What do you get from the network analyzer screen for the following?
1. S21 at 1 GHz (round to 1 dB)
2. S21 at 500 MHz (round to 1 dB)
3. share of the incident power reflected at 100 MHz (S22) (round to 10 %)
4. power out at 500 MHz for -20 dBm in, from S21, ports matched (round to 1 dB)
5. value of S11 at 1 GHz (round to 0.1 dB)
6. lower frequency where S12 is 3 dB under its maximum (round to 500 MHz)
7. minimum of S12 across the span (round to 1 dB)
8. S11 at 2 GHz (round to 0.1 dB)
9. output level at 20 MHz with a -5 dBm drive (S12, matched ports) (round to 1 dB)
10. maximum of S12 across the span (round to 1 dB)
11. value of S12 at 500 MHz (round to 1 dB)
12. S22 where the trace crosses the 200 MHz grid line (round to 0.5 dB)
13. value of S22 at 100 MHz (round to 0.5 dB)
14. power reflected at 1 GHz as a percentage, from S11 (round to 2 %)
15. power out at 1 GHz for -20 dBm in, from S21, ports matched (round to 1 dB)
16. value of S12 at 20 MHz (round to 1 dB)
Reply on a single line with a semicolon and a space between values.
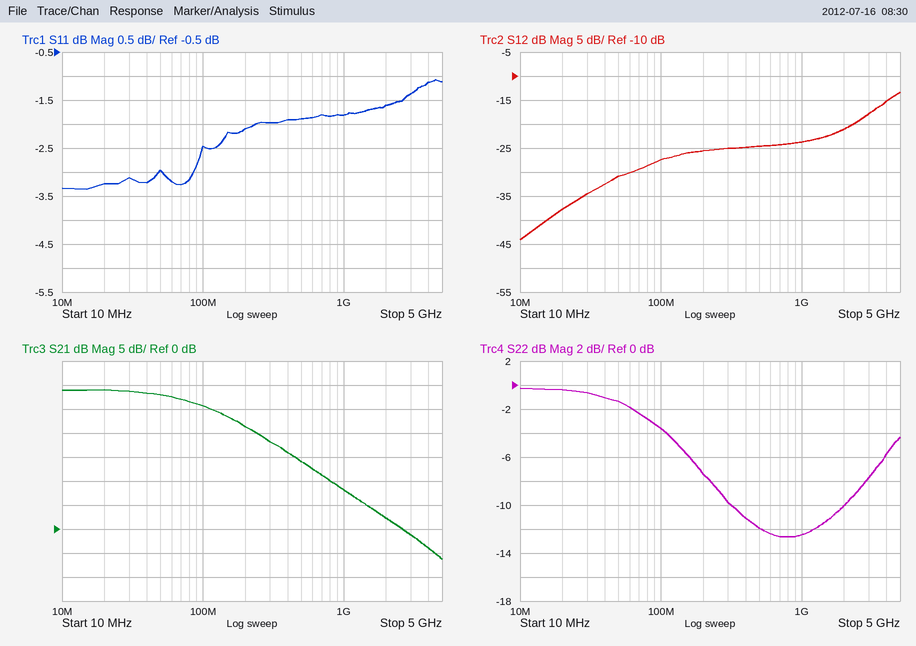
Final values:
8 dB; 14 dB; 40 %; -6 dBm; -1.8 dB; 3.5 GHz; -44 dB; -1.6 dB; -43 dBm; -13 dB; -25 dB; -7.5 dB; -3.5 dB; 66 %; -12 dBm; -38 dB
